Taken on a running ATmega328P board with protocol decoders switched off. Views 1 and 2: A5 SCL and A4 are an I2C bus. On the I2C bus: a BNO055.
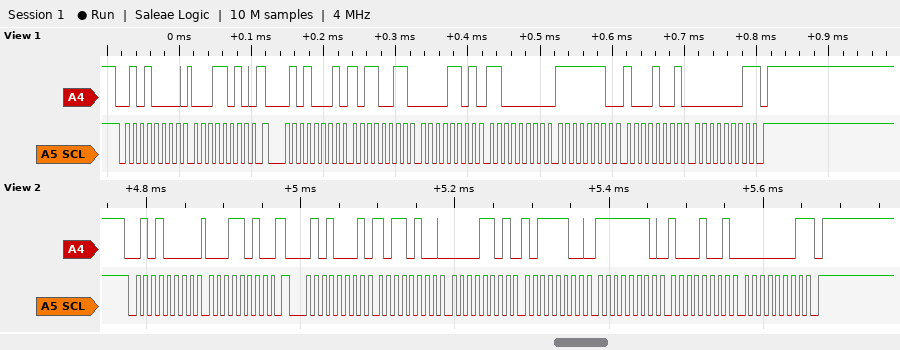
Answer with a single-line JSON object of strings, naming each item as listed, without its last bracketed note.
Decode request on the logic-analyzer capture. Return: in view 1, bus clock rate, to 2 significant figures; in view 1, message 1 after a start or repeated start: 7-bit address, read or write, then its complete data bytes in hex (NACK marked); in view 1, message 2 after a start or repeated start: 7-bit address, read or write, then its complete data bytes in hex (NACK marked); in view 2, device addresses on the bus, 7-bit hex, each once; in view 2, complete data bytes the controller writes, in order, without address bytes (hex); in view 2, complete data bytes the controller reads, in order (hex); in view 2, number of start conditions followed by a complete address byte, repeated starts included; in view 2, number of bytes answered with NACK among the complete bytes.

{"in view 1, bus clock rate, to 2 significant figures": "100 kHz", "in view 1, message 1 after a start or repeated start: 7-bit address, read or write, then its complete data bytes in hex": "0x28 write: 1A", "in view 1, message 2 after a start or repeated start: 7-bit address, read or write, then its complete data bytes in hex": "0x28 read: B3 0D C0 FE 89 01 NACK", "in view 2, device addresses on the bus, 7-bit hex, each once": "0x28", "in view 2, complete data bytes the controller writes, in order, without address bytes": "1A", "in view 2, complete data bytes the controller reads, in order": "B4 0D BC FE 89 01", "in view 2, number of start conditions followed by a complete address byte, repeated starts included": "2", "in view 2, number of bytes answered with NACK among the complete bytes": "1"}
